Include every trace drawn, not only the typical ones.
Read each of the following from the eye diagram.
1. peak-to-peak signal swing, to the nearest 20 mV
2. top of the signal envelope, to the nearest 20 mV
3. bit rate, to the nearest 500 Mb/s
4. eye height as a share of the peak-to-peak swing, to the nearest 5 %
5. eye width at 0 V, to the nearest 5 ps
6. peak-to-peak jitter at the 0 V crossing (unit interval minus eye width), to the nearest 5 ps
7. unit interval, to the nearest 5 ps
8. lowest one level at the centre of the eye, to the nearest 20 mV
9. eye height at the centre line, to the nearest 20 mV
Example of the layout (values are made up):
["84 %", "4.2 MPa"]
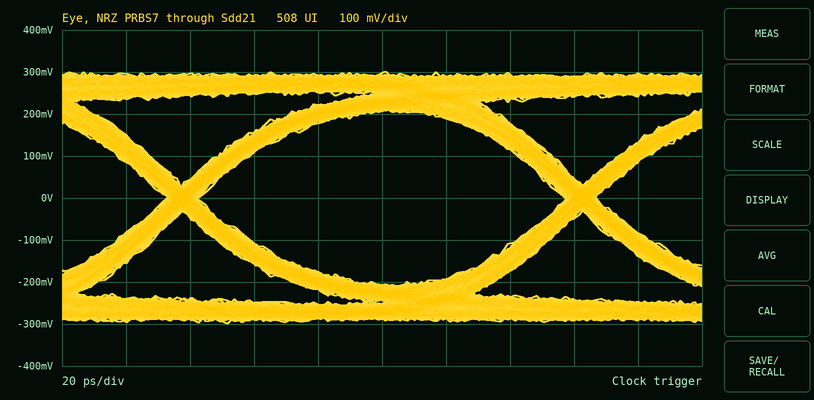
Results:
["600 mV", "300 mV", "8.0 Gb/s", "70 %", "115 ps", "10 ps", "125 ps", "200 mV", "420 mV"]
